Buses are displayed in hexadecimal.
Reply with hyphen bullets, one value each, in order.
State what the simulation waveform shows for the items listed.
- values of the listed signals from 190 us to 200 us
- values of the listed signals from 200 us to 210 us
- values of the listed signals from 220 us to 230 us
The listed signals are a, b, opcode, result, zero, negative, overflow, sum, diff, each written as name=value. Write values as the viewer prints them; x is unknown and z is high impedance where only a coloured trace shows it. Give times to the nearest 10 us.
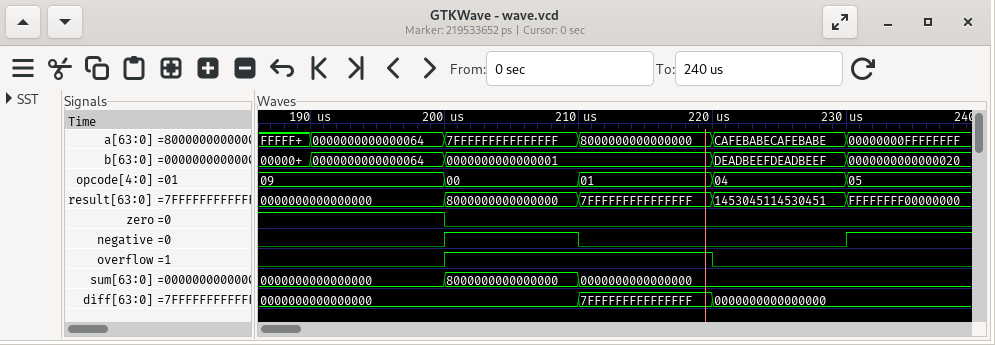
- a=0000000000000064, b=0000000000000064, opcode=09, result=0000000000000000, zero=1, negative=0, overflow=0, sum=0000000000000000, diff=0000000000000000
- a=7FFFFFFFFFFFFFFF, b=0000000000000001, opcode=00, result=8000000000000000, zero=0, negative=1, overflow=1, sum=8000000000000000, diff=0000000000000000
- a=CAFEBABECAFEBABE, b=DEADBEEFDEADBEEF, opcode=04, result=1453045114530451, zero=0, negative=0, overflow=0, sum=0000000000000000, diff=0000000000000000
